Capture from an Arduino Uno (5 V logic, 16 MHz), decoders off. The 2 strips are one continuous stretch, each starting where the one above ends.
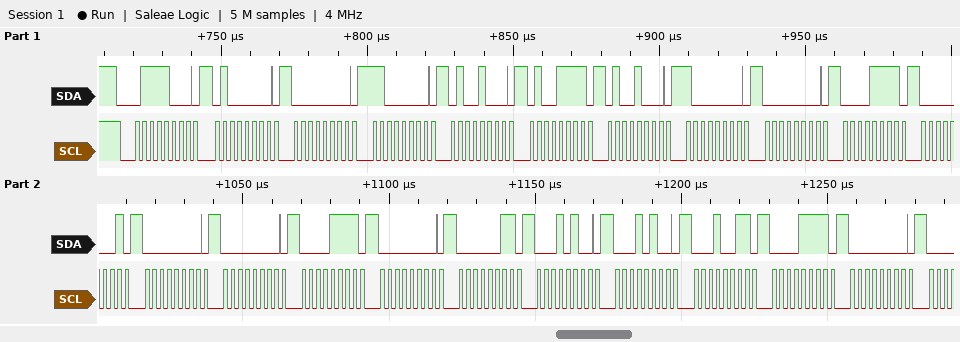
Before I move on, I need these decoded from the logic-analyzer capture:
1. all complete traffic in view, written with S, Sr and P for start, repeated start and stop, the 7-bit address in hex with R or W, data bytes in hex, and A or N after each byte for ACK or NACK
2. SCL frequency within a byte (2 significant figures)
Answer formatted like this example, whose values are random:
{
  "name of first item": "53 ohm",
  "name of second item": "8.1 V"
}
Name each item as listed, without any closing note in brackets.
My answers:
{
  "all complete traffic in view, written with S, Sr and P for start, repeated start and stop, the 7-bit address in hex with R or W, data bytes in hex, and A or N after each byte for ACK or NACK": "S 3CW A 40 A 00 A C0 A 48 A 4F A 48 A 80 A 00 A 0F A 01 A 00 A 00 A 0F A 00 A 03 A 14 A 14 A 13 A 0F A 00 A",
  "SCL frequency within a byte": "400 kHz"
}
